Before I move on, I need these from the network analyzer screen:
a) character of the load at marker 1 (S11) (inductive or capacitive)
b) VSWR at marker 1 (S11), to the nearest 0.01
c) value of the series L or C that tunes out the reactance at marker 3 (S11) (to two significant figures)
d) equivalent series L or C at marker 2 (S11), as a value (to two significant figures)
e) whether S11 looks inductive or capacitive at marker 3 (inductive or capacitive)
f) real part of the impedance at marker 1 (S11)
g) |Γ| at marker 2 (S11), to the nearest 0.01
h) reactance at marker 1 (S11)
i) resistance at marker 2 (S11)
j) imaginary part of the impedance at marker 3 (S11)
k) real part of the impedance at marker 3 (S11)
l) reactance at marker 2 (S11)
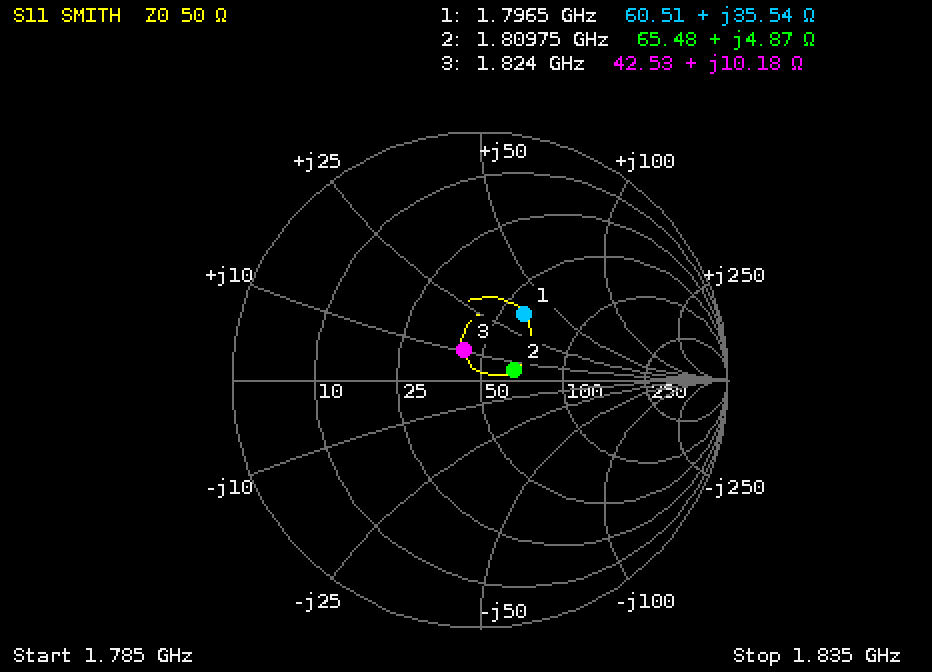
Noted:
inductive
1.94
8.6 pF
430 pH
inductive
60.51 Ω
0.14
+35.54 Ω
65.48 Ω
+10.18 Ω
42.53 Ω
+4.87 Ω
